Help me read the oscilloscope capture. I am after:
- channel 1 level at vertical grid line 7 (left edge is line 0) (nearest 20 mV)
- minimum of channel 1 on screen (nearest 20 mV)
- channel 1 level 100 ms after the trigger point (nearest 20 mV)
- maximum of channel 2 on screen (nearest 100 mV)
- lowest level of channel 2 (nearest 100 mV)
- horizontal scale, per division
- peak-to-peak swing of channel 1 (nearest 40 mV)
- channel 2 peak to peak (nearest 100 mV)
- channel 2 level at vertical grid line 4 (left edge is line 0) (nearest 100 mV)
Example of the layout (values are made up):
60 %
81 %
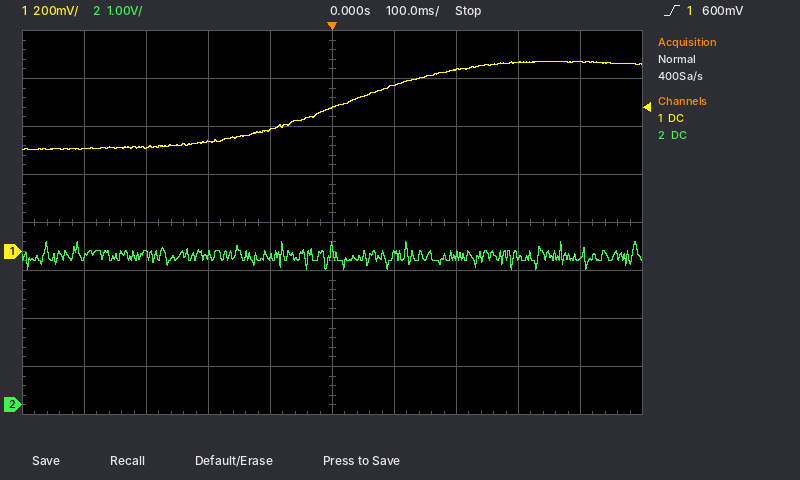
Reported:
760 mV
420 mV
700 mV
3.4 V
2.8 V
100 ms
360 mV
600 mV
3.1 V
